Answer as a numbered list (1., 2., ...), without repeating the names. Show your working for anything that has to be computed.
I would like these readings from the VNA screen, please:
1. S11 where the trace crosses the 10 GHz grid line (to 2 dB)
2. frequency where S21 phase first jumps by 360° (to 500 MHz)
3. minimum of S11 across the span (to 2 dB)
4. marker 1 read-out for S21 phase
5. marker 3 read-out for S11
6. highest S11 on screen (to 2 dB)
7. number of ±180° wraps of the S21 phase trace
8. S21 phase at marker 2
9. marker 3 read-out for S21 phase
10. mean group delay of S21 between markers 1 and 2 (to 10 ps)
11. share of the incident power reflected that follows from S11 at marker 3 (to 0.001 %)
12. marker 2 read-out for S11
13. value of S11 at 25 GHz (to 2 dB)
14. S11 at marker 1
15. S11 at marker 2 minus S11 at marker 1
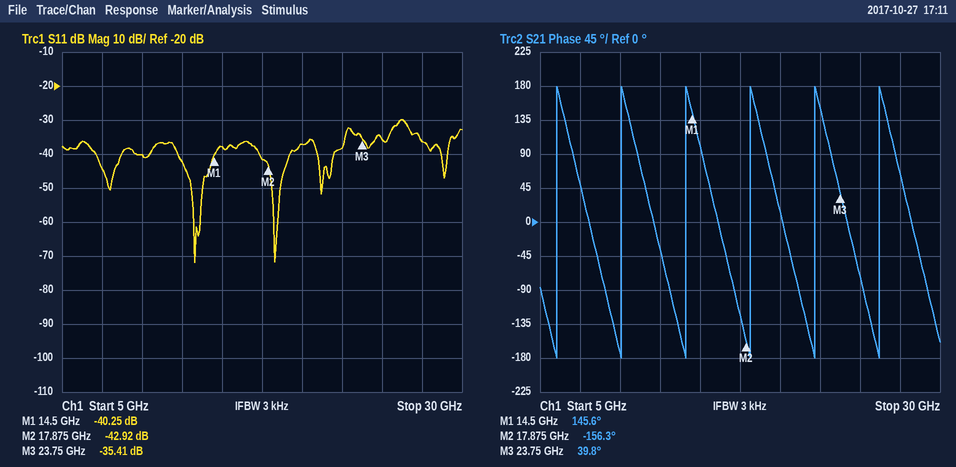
1. -40 dB
2. 6.0 GHz
3. -72 dB
4. 145.6°
5. -35.41 dB
6. -30 dB
7. 6
8. -156.3°
9. 39.8°
10. −(-156.3° − (145.6°))/(360° × 3.375 GHz) ≈ 248 ps, so 250 ps to the nearest 10 ps
11. 10^(-35.41/10) ≈ 0.029 %
12. -42.92 dB
13. -36 dB
14. -40.25 dB
15. -42.92 − (-40.25) = -2.67 dB
